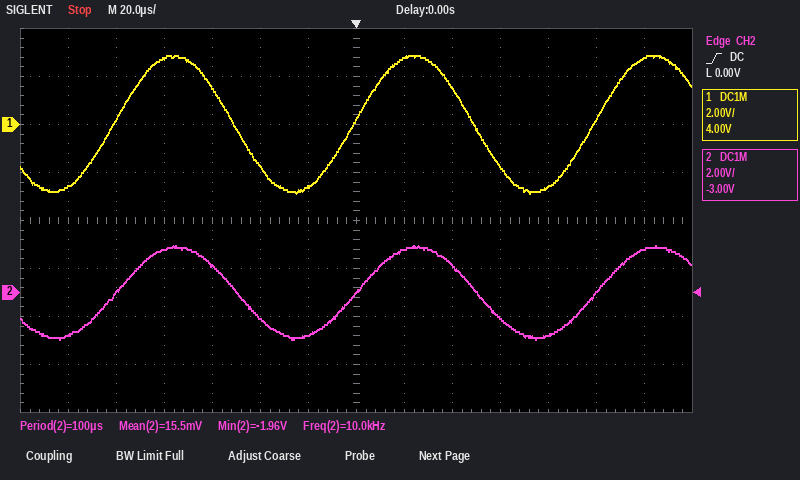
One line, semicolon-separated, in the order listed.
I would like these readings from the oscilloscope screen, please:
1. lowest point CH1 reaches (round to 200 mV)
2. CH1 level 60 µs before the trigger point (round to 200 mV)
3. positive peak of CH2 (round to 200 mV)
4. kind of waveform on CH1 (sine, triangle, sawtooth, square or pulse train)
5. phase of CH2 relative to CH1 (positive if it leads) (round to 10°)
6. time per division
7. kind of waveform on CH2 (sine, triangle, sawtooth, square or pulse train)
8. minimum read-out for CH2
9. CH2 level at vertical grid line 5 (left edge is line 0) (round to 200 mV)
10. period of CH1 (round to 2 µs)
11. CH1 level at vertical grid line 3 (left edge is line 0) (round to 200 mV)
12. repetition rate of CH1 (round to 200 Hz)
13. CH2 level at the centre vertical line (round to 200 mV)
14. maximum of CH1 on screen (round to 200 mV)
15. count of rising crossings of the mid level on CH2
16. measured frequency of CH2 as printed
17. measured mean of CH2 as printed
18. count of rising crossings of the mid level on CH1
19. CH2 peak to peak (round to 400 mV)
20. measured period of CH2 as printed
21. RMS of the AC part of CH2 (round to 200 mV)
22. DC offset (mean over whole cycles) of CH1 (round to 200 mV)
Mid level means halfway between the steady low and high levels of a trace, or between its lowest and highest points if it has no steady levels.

-2.8 V; 1.6 V; 2.0 V; sine; 0°; 20 µs; sine; -1.96 V; -1.0 V; 100 µs; 2.8 V; 10.0 kHz; 0.0 V; 2.8 V; 3; 10.0 kHz; 15.5 mV; 3; 4.0 V; 100 µs; 1.4 V; 0.0 V
